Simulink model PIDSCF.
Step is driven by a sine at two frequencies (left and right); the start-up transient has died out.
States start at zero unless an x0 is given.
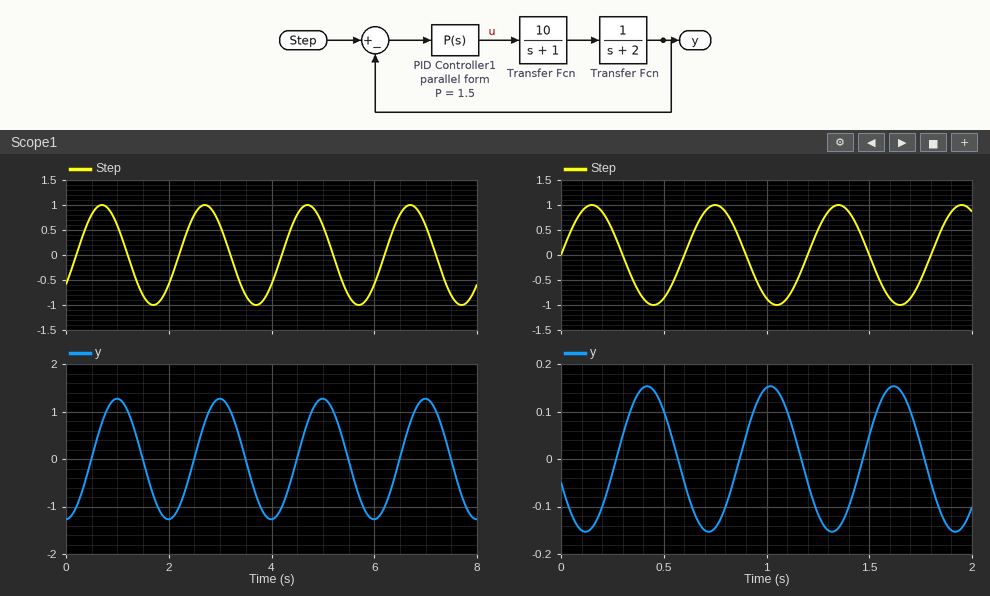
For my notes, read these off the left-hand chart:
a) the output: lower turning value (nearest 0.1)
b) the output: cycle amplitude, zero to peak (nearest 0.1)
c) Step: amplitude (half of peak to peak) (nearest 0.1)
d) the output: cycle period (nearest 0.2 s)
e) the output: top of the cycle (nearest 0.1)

-1.3
1.3
1.0
2.0 s
1.3
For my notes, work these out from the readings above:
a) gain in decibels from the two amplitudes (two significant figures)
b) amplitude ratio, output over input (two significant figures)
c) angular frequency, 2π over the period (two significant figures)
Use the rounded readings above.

2.3 dB
1.3
3.1 rad/s
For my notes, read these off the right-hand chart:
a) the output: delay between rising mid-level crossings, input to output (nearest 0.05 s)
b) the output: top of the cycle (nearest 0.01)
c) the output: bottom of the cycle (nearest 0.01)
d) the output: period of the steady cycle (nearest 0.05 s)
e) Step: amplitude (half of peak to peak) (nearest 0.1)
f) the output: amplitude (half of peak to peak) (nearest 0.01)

0.25 s
0.15
-0.15
0.60 s
1.0
0.15
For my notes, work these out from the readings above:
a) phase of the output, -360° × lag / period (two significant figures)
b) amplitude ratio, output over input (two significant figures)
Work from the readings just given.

-150°
0.15
